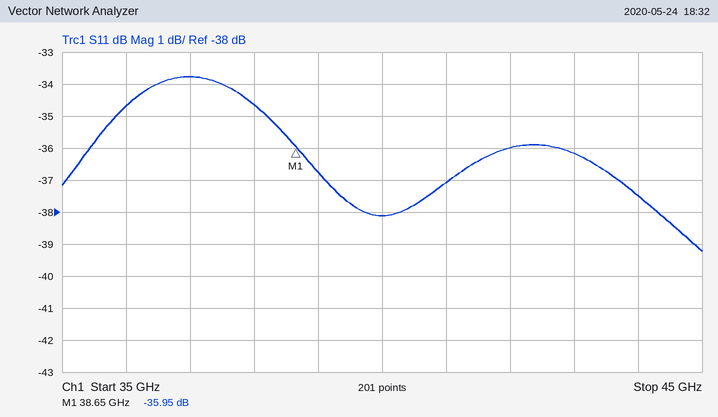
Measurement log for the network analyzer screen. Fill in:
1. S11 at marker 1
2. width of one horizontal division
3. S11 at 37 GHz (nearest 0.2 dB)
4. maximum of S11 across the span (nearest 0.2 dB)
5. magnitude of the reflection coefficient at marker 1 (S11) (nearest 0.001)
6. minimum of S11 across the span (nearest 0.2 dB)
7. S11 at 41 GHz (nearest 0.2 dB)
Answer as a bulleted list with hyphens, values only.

- -35.95 dB
- 1 GHz
- -33.8 dB
- -33.8 dB
- 0.016
- -39.2 dB
- -37.0 dB
